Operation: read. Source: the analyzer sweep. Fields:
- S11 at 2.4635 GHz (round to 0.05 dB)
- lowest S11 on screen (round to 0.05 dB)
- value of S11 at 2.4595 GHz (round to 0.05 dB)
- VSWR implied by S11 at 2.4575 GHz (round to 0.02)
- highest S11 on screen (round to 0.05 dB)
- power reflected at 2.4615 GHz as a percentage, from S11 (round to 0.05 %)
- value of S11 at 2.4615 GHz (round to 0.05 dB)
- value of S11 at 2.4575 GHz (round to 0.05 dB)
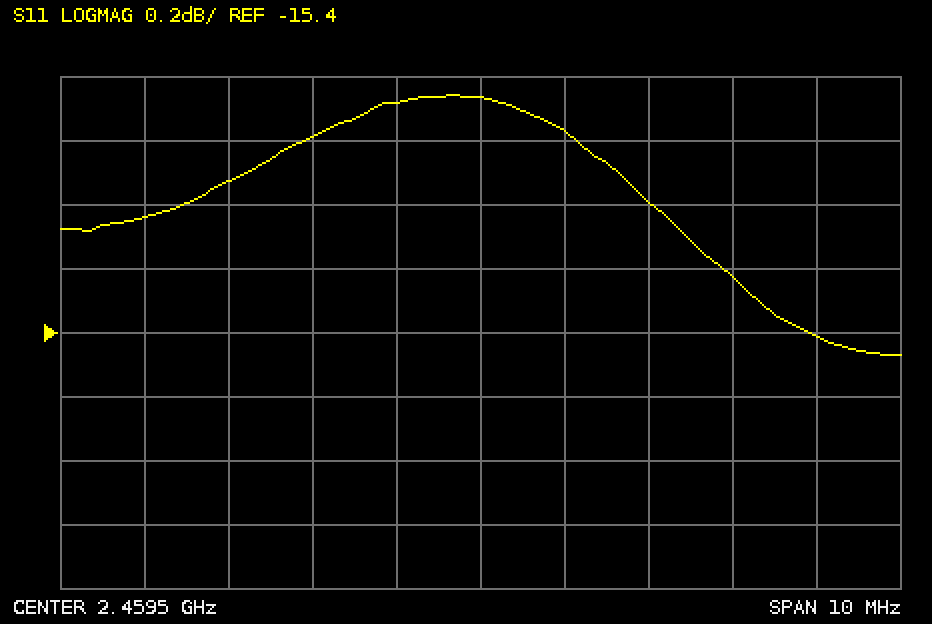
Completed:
-15.40 dB
-15.45 dB
-14.65 dB
1.44
-14.65 dB
3.15 %
-15.00 dB
-14.80 dB
